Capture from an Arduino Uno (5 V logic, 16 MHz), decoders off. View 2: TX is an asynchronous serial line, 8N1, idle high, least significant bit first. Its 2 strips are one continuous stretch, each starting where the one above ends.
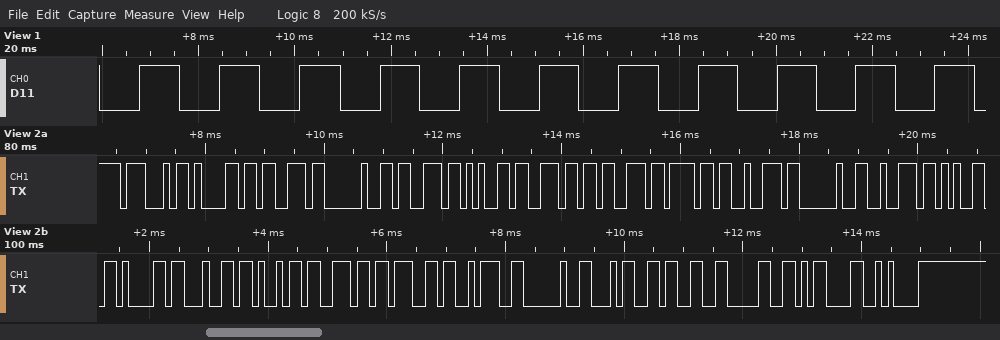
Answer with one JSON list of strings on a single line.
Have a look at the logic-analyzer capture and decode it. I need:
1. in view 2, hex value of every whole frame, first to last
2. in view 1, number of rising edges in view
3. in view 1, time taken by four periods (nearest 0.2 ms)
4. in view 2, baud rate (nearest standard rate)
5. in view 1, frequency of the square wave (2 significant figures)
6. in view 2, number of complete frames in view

["47 61 73 20 73 65 6E 73 6F 72 20 72 65 61 64 69 6E 67 3A 20 34 33 30 0D 0A", "11", "6.6 ms", "9600 baud", "610 Hz", "25"]
